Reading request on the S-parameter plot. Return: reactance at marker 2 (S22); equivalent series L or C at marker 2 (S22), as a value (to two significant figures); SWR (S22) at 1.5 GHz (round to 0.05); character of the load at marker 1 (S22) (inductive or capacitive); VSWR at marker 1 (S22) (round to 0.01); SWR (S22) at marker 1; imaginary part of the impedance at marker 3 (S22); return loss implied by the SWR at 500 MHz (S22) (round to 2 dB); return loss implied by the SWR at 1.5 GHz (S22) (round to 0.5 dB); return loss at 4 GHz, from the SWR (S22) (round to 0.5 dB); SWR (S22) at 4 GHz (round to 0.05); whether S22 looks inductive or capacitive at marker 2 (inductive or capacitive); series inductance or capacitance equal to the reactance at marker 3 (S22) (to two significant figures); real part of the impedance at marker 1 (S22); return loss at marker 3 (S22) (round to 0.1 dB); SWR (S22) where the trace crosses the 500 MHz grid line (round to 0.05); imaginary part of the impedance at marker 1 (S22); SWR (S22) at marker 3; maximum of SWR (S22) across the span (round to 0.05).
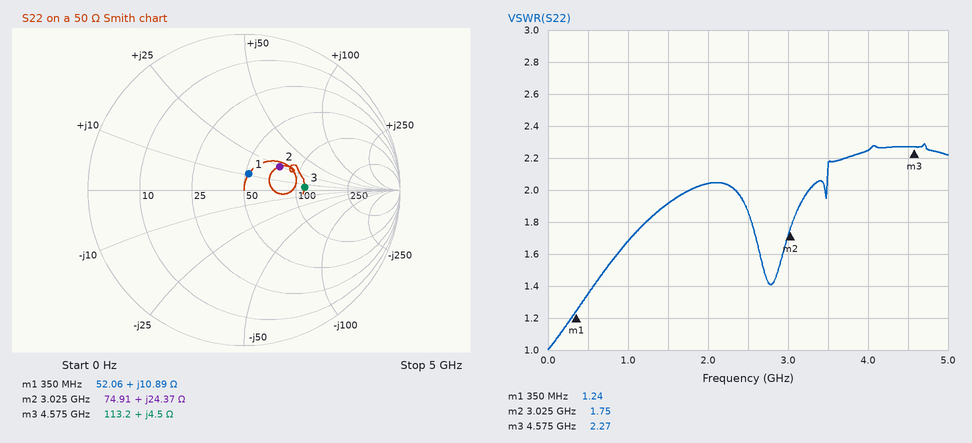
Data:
+24.37 Ω
1.3 nH
1.90
inductive
1.24
1.24
+4.5 Ω
16 dB
10.0 dB
8.5 dB
2.25
inductive
160 pH
52.06 Ω
8.2 dB
1.35
+10.89 Ω
2.27
2.30
